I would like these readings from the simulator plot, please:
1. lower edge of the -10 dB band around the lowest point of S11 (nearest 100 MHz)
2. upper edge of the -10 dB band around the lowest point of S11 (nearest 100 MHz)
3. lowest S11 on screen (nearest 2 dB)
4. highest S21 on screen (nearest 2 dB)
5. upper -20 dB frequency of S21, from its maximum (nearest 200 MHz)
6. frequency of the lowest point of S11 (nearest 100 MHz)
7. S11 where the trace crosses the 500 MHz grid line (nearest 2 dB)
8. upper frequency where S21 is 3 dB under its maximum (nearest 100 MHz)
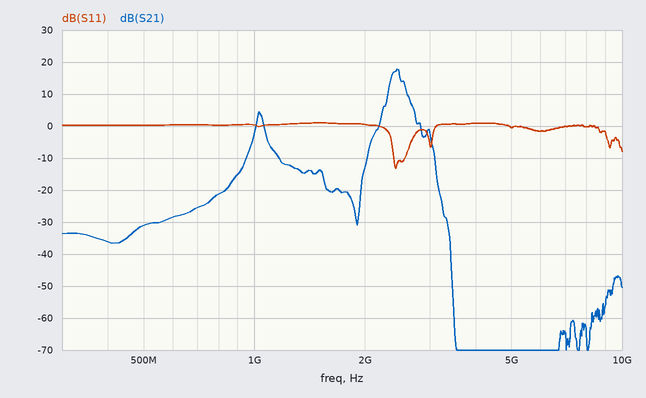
2.4 GHz
2.6 GHz
-14 dB
18 dB
2.8 GHz
2.4 GHz
0 dB
2.5 GHz
